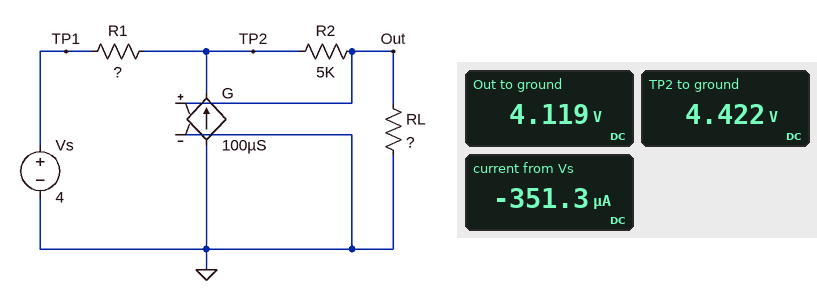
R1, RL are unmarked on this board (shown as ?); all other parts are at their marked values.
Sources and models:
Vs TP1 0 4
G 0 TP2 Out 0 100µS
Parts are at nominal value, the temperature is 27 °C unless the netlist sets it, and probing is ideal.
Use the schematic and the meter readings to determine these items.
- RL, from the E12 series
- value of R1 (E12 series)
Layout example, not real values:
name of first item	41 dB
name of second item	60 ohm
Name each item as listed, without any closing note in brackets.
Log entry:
RL, from the E12 series	68 kΩ
value of R1	1.2 kΩ
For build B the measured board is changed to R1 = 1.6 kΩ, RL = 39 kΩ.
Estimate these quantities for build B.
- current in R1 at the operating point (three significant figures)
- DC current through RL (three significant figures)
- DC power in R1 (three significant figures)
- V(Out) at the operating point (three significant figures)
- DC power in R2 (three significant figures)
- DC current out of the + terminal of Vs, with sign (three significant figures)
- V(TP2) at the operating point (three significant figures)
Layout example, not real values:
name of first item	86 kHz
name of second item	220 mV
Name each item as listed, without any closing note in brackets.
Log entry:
current in R1 at the operating point	295 µA
DC current through RL	102 µA
DC power in R1	139 µW
V(Out) at the operating point	3.96 V
DC power in R2	51.6 µW
DC current out of the + terminal of Vs, with sign	-295 µA
V(TP2) at the operating point	4.47 V
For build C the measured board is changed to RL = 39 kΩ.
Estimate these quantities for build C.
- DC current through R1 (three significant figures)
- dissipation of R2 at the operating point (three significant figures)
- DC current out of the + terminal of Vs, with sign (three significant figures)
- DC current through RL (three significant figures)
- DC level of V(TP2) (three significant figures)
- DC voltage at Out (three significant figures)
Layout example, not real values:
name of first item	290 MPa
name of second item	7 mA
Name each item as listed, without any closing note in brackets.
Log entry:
DC current through R1	286 µA
dissipation of R2 at the operating point	48.7 µW
DC current out of the + terminal of Vs, with sign	-286 µA
DC current through RL	98.7 µA
DC level of V(TP2)	4.34 V
DC voltage at Out	3.85 V
